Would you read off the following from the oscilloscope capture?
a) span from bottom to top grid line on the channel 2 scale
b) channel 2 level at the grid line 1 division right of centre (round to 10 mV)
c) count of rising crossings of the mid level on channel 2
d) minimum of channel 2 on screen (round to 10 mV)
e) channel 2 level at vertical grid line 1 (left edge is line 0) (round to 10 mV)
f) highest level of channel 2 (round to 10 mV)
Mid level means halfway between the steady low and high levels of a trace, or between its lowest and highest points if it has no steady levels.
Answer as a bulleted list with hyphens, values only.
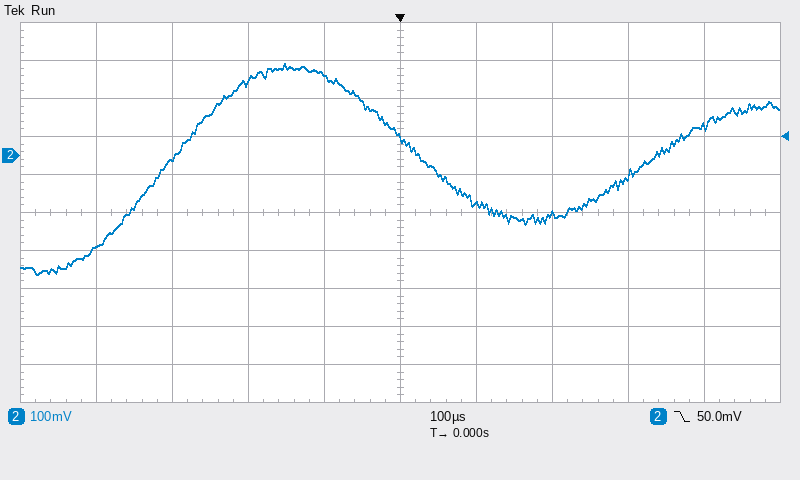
- 1 V
- -130 mV
- 2
- -310 mV
- -240 mV
- 240 mV
